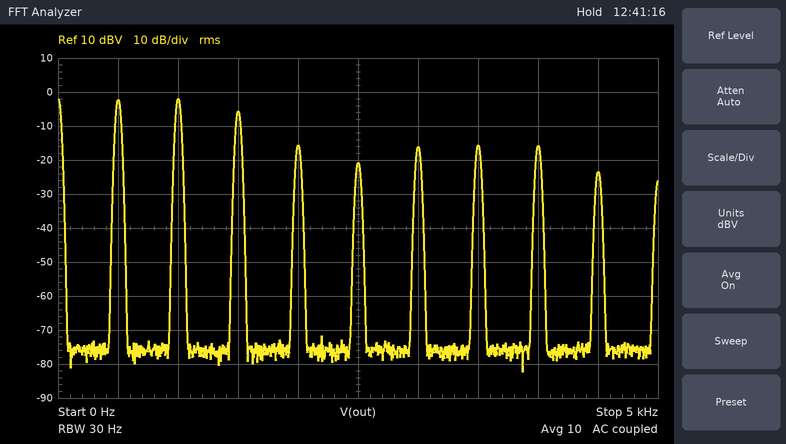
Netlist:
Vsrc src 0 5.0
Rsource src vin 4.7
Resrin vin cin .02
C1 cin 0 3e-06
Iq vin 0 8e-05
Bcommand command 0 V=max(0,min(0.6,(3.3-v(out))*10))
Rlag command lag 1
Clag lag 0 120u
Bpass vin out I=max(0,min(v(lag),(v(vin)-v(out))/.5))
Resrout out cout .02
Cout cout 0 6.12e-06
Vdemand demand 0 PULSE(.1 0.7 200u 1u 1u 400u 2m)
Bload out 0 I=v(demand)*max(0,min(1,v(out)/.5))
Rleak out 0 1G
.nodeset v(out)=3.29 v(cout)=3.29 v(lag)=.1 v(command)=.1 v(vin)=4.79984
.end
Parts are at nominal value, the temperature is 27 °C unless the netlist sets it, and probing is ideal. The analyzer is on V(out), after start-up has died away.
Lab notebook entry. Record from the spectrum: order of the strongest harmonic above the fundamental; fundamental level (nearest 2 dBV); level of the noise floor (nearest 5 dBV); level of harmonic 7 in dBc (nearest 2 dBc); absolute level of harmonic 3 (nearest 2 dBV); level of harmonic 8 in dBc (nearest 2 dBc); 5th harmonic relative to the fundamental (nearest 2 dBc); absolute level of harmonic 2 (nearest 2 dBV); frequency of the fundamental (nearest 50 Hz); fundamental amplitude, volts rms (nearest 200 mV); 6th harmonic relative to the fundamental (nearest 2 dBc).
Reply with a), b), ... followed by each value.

a) 2
b) -2 dBV
c) -75 dBV
d) -14 dBc
e) -6 dBV
f) -14 dBc
g) -18 dBc
h) -2 dBV
i) 500 Hz
j) 800 mV
k) -14 dBc
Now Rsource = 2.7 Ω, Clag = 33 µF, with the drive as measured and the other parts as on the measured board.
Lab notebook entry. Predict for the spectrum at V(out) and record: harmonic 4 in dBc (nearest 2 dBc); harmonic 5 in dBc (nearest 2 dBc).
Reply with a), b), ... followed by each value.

a) -8 dBc
b) -20 dBc
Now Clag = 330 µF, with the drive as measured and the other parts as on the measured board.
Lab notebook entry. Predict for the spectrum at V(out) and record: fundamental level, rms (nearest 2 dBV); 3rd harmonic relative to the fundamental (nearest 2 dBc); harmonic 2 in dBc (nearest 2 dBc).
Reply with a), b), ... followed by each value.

a) 0 dBV
b) -8 dBc
c) -2 dBc
